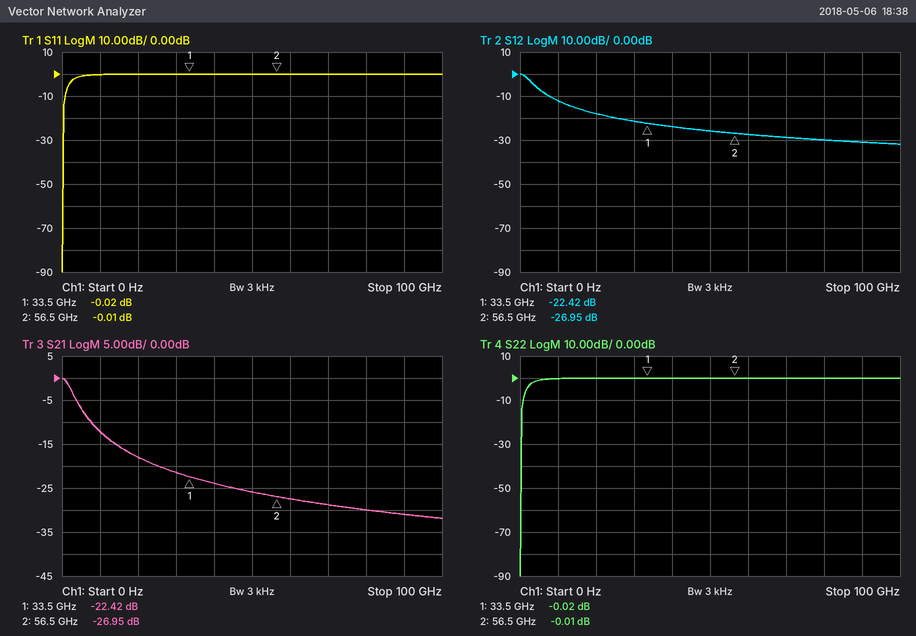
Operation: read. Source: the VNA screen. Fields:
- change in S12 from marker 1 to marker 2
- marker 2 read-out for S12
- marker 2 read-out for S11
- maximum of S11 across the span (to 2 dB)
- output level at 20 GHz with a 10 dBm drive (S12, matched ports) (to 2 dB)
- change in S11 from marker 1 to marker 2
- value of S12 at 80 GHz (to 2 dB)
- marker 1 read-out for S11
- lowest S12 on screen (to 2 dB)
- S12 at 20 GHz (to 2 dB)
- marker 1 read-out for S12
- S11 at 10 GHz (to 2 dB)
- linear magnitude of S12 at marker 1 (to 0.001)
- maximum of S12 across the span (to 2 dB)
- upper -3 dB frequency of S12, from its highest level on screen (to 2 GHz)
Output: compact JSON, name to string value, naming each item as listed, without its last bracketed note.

{"change in S12 from marker 1 to marker 2": "-4.53 dB", "marker 2 read-out for S12": "-26.95 dB", "marker 2 read-out for S11": "-0.01 dB", "maximum of S11 across the span": "0 dB", "output level at 20 GHz with a 10 dBm drive (S12, matched ports)": "-8 dBm", "change in S11 from marker 1 to marker 2": "0.01 dB", "value of S12 at 80 GHz": "-30 dB", "marker 1 read-out for S11": "-0.02 dB", "lowest S12 on screen": "-32 dB", "S12 at 20 GHz": "-18 dB", "marker 1 read-out for S12": "-22.42 dB", "S11 at 10 GHz": "0 dB", "linear magnitude of S12 at marker 1": "0.076", "maximum of S12 across the span": "0 dB", "upper -3 dB frequency of S12, from its highest level on screen": "2 GHz"}
